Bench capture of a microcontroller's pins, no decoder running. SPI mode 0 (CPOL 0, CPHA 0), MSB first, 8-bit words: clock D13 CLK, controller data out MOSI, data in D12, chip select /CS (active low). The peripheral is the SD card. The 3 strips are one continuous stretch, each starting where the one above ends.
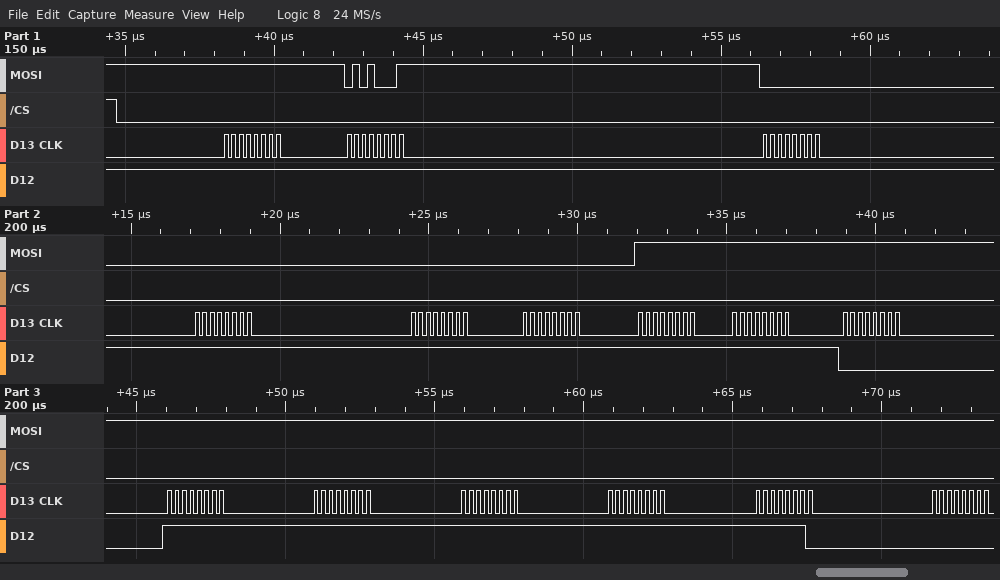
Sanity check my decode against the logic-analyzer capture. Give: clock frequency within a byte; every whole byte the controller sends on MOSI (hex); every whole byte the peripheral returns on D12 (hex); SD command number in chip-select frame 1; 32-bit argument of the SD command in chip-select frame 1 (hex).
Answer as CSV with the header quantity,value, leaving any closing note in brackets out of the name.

quantity,value
clock frequency within a byte,4 MHz
every whole byte the controller sends on MOSI,0xFF 0x51 0x00 0x00 0x00 0x00 0xFF 0xFF 0xFF 0xFF 0xFF 0xFF 0xFF 0xFF 0xFF
every whole byte the peripheral returns on D12,0xFF 0xFF 0xFF 0xFF 0xFF 0xFF 0xFF 0xFF 0x00 0xFF 0xFF 0xFF 0xFF 0xFE 0x00
SD command number in chip-select frame 1,CMD17
32-bit argument of the SD command in chip-select frame 1,0x00000000
